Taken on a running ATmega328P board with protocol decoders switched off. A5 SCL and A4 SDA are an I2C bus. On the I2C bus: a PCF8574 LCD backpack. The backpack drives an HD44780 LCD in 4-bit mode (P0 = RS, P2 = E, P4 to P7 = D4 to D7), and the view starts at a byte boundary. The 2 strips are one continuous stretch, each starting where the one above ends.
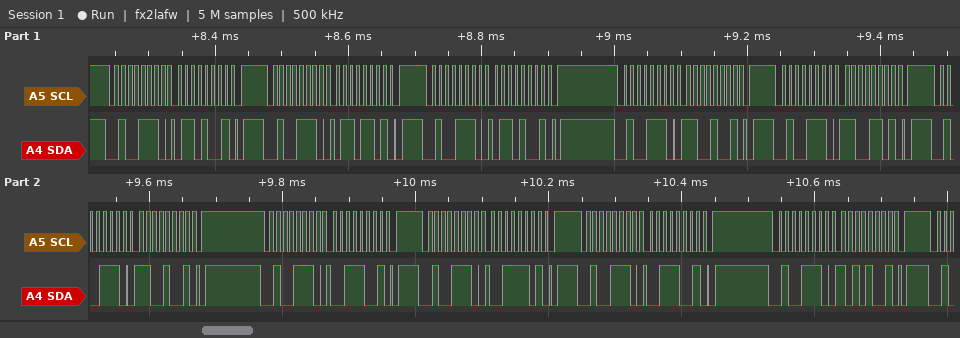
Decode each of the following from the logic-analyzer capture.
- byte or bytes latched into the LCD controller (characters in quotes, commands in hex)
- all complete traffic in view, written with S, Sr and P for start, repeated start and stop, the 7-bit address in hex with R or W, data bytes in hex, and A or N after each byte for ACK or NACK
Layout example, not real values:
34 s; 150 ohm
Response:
'l'; S 27W A 69 A P S 27W A 6D A P S 27W A 69 A P S 27W A C9 A P S 27W A CD A P S 27W A C9 A P S 27W A 39 A P S 27W A 3D A P S 27W A 39 A P S 27W A A9 A P
